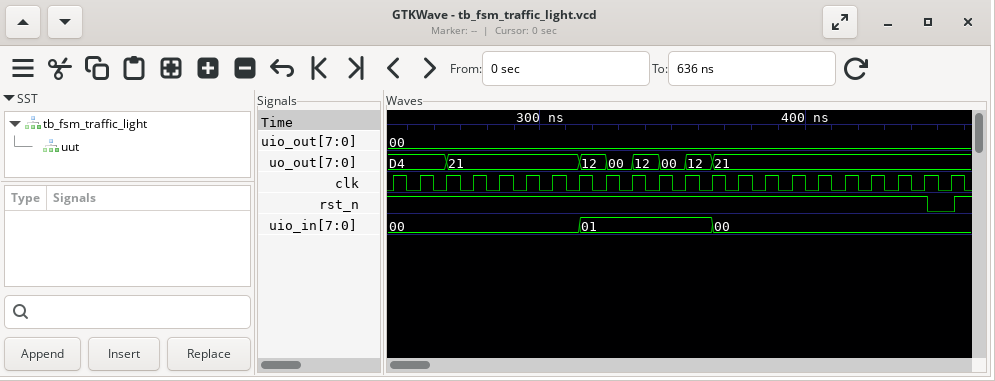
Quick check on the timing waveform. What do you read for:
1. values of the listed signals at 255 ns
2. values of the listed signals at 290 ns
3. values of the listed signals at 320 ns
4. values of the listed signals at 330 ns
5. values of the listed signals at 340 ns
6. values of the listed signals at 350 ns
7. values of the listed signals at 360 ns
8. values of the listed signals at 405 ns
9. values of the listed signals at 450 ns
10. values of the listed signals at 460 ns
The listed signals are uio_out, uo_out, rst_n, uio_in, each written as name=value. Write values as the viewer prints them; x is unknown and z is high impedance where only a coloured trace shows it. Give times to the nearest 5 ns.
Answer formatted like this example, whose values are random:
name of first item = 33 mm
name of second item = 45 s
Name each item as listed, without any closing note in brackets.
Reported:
values of the listed signals at 255 ns = uio_out=00, uo_out=D4, rst_n=1, uio_in=00
values of the listed signals at 290 ns = uio_out=00, uo_out=21, rst_n=1, uio_in=00
values of the listed signals at 320 ns = uio_out=00, uo_out=12, rst_n=1, uio_in=01
values of the listed signals at 330 ns = uio_out=00, uo_out=00, rst_n=1, uio_in=01
values of the listed signals at 340 ns = uio_out=00, uo_out=12, rst_n=1, uio_in=01
values of the listed signals at 350 ns = uio_out=00, uo_out=00, rst_n=1, uio_in=01
values of the listed signals at 360 ns = uio_out=00, uo_out=12, rst_n=1, uio_in=01
values of the listed signals at 405 ns = uio_out=00, uo_out=21, rst_n=1, uio_in=00
values of the listed signals at 450 ns = uio_out=00, uo_out=21, rst_n=0, uio_in=00
values of the listed signals at 460 ns = uio_out=00, uo_out=21, rst_n=1, uio_in=00
